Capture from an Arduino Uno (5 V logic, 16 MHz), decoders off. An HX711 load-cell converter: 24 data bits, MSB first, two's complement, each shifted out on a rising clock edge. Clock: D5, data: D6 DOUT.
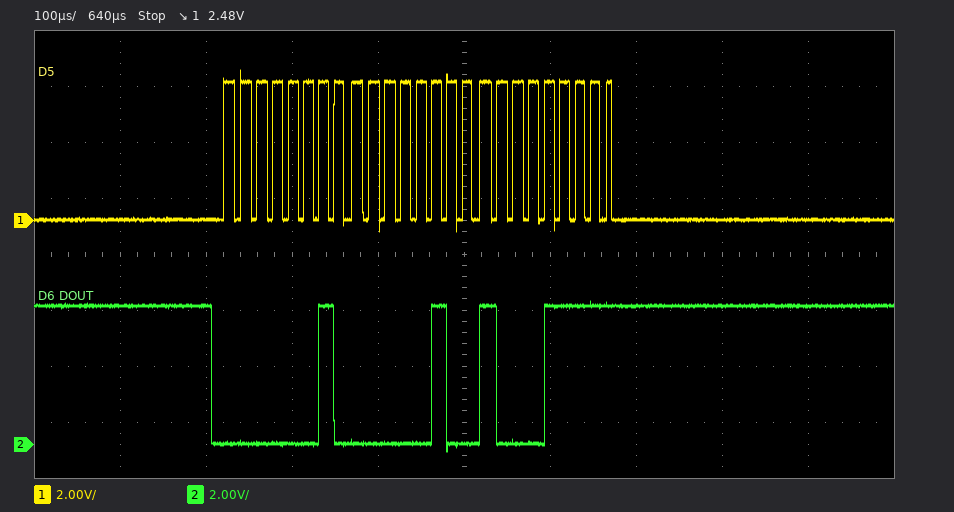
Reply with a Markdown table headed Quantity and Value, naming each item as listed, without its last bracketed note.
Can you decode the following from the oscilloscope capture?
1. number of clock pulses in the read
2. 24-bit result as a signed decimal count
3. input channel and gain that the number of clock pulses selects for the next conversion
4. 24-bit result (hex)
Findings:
| Quantity | Value |
|---|---|
| number of clock pulses in the read | 25 |
| 24-bit result as a signed decimal count | 132239 |
| input channel and gain that the number of clock pulses selects for the next conversion | channel A, gain 128 |
| 24-bit result | 0x02048F |
